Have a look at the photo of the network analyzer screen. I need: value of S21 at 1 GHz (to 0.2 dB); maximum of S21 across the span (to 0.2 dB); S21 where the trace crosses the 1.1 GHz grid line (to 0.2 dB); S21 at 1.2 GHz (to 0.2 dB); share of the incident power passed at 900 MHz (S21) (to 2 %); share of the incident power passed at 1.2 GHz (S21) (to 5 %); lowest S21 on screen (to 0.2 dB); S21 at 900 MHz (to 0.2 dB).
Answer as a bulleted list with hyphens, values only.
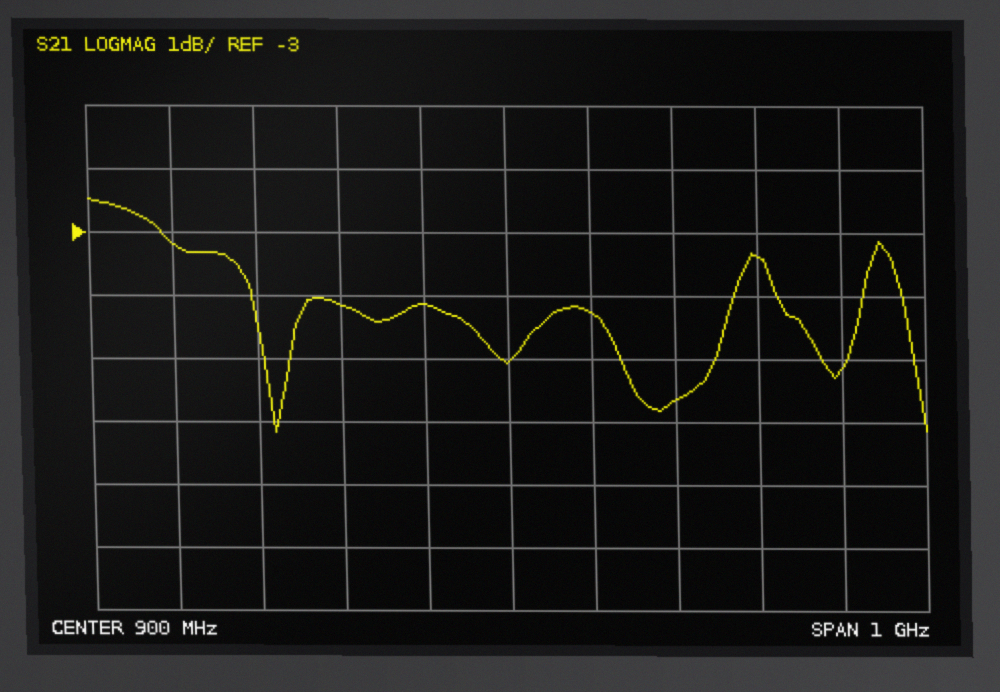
- -4.2 dB
- -2.4 dB
- -5.6 dB
- -3.4 dB
- 32 %
- 45 %
- -6.2 dB
- -5.0 dB
